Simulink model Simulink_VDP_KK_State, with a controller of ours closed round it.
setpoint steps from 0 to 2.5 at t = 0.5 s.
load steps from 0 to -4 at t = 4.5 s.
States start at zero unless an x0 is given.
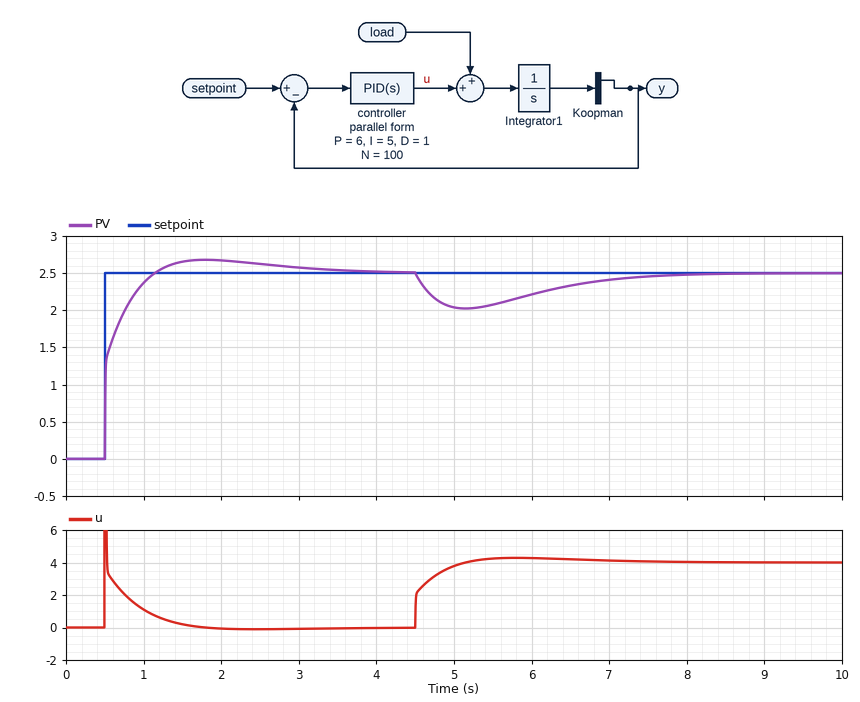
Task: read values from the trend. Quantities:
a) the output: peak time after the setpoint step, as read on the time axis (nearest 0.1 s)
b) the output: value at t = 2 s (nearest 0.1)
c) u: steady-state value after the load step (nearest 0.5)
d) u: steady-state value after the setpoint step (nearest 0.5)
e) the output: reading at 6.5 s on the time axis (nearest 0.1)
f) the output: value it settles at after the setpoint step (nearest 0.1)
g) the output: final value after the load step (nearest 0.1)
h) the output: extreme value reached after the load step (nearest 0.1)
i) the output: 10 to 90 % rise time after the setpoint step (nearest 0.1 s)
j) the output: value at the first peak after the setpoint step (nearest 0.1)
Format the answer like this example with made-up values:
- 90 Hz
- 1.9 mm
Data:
- 1.8 s
- 2.7
- 4.0
- 0.0
- 2.3
- 2.5
- 2.5
- 2.0
- 0.4 s
- 2.7
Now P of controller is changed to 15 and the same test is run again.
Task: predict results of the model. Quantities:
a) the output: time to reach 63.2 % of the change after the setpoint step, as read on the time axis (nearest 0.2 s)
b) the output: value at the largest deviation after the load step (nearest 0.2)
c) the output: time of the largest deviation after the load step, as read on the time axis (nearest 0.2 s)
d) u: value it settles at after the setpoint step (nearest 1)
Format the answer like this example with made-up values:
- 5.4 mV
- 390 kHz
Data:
- 0.6 s
- 2.2
- 5.0 s
- 0
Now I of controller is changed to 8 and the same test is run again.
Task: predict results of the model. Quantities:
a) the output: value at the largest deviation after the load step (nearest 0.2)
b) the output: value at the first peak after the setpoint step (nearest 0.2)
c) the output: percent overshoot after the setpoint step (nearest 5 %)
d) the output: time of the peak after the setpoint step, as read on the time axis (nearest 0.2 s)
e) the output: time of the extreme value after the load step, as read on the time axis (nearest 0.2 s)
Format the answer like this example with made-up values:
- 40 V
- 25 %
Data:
- 2.0
- 2.8
- 10 %
- 1.6 s
- 5.0 s
